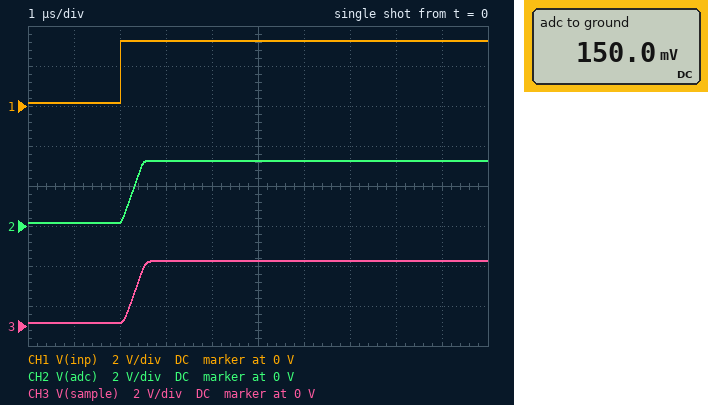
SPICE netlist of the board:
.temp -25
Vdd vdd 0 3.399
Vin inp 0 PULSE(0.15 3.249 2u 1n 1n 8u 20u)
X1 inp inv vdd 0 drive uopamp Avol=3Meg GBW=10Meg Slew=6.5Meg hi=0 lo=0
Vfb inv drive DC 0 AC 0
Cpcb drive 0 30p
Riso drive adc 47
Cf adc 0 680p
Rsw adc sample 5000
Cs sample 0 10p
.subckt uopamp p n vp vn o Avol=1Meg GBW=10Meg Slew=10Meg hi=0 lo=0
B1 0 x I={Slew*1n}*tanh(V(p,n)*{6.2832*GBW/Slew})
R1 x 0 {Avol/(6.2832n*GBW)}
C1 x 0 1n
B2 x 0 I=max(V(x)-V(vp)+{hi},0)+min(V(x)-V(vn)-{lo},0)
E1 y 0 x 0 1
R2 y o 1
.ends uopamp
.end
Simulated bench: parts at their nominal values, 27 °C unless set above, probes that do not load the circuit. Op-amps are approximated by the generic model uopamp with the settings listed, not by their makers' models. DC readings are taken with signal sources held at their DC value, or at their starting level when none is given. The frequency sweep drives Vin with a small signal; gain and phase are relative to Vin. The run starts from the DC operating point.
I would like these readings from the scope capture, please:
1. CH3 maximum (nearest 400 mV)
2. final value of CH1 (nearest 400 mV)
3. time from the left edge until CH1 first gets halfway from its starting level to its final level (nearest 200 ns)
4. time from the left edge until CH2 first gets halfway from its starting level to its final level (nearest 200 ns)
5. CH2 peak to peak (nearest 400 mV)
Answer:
3.2 V
3.2 V
2.0 µs
2.2 µs
3.2 V
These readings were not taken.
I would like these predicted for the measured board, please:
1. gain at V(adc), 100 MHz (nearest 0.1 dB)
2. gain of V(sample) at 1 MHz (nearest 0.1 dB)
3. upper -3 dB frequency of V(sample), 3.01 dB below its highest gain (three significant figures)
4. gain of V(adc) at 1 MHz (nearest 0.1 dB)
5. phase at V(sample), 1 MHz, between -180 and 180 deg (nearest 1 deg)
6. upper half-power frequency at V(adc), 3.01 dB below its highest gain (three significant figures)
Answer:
-46.3 dB
-0.6 dB
2.35 MHz
-0.2 dB
-35 deg
4.15 MHz
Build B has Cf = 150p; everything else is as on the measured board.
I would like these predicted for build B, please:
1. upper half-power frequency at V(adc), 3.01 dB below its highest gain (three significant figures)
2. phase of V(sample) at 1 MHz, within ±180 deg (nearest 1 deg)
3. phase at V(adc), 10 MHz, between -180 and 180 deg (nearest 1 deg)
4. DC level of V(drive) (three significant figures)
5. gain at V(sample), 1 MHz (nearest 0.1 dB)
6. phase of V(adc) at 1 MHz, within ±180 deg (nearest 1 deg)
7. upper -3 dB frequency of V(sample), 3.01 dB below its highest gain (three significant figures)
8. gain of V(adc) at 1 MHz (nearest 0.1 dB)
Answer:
8.55 MHz
-26 deg
-69 deg
150 mV
-0.5 dB
-8 deg
2.86 MHz
-0.1 dB
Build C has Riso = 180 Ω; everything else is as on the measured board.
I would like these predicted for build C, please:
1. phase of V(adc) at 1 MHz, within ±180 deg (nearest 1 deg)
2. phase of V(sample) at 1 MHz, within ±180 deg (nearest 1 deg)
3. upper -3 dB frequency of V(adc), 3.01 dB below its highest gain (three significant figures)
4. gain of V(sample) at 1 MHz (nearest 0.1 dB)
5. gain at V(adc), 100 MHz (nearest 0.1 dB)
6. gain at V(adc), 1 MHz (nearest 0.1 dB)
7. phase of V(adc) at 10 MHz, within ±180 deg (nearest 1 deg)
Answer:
-44 deg
-61 deg
1.26 MHz
-2.5 dB
-57.8 dB
-2.1 dB
-128 deg
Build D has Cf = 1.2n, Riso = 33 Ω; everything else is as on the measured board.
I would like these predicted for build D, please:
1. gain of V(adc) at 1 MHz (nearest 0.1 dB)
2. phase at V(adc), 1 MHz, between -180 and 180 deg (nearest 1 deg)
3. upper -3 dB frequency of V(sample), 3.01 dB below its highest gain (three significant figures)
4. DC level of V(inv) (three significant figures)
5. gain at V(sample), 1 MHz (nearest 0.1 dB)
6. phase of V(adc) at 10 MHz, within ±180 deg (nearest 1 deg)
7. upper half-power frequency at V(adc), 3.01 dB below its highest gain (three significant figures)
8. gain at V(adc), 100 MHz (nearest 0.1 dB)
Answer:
-0.3 dB
-20 deg
2.19 MHz
150 mV
-0.7 dB
-114 deg
3.54 MHz
-48.2 dB
